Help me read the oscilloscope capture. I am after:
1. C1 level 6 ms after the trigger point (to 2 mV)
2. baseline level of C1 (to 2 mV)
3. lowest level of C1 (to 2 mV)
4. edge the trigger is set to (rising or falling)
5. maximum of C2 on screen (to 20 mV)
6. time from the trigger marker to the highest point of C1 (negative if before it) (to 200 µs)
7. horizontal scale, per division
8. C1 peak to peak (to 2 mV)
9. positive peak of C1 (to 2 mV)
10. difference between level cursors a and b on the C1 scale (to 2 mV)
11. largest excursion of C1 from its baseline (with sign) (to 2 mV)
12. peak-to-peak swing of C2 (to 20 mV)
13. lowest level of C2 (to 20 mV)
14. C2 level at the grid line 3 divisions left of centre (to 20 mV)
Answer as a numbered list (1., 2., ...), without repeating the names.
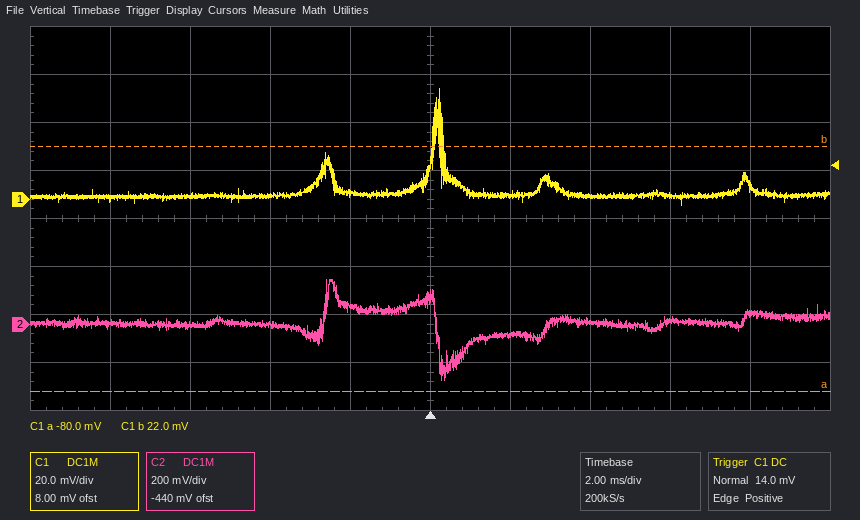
1. 2 mV
2. 2 mV
3. -2 mV
4. rising
5. 180 mV
6. +200 µs
7. 2 ms
8. 48 mV
9. 46 mV
10. 102 mV
11. +44 mV
12. 420 mV
13. -240 mV
14. 0 mV
